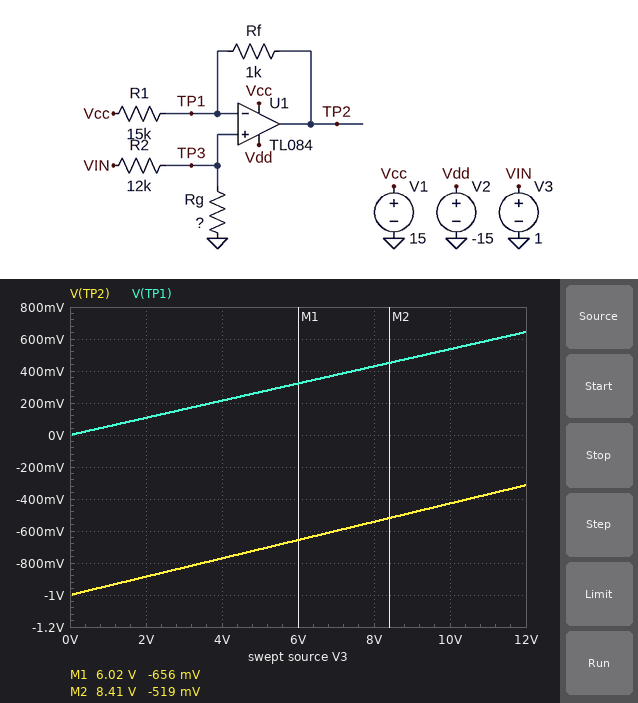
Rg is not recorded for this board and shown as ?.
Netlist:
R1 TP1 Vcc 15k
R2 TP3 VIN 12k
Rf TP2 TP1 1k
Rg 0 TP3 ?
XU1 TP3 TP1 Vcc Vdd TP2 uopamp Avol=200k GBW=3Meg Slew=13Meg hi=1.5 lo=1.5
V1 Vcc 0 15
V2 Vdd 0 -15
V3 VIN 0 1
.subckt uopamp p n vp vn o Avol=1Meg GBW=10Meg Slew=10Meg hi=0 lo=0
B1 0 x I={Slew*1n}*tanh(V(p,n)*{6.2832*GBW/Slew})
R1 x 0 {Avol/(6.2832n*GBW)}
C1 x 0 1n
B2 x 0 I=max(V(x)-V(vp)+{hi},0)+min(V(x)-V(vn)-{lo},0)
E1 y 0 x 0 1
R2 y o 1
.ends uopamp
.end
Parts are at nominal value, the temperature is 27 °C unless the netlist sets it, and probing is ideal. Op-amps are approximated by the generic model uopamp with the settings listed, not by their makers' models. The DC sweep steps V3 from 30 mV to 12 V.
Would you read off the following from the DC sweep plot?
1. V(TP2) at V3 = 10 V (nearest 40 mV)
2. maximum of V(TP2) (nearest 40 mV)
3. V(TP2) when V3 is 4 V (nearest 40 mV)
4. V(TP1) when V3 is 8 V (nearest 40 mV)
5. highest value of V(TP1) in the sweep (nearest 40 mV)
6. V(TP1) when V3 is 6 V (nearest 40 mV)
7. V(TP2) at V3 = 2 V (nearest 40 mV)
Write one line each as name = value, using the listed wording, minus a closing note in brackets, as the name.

V(TP2) at V3 = 10 V = -440 mV
maximum of V(TP2) = -320 mV
V(TP2) when V3 is 4 V = -760 mV
V(TP1) when V3 is 8 V = 440 mV
highest value of V(TP1) in the sweep = 640 mV
V(TP1) when V3 is 6 V = 320 mV
V(TP2) at V3 = 2 V = -880 mV
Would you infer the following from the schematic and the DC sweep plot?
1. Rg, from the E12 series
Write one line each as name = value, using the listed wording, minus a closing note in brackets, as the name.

Rg, from the E12 series = 680 Ω
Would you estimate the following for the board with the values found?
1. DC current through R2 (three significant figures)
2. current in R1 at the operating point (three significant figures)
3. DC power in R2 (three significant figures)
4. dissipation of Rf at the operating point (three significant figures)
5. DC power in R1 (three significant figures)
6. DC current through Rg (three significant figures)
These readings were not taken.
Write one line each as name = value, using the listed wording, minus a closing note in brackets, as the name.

DC current through R2 = 78.9 µA
current in R1 at the operating point = 996 µA
DC power in R2 = 74.6 µW
dissipation of Rf at the operating point = 993 µW
DC power in R1 = 14.9 mW
DC current through Rg = 78.9 µA
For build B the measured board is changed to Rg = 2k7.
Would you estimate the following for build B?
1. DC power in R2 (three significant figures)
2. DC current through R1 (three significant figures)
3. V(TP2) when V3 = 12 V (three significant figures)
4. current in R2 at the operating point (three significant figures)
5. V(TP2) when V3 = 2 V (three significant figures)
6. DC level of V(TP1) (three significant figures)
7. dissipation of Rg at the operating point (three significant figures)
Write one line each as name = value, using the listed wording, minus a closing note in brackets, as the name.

DC power in R2 = 55.5 µW
DC current through R1 = 988 µA
V(TP2) when V3 = 12 V = 1.35 V
current in R2 at the operating point = 68.0 µA
V(TP2) when V3 = 2 V = -608 mV
DC level of V(TP1) = 184 mV
dissipation of Rg at the operating point = 12.5 µW
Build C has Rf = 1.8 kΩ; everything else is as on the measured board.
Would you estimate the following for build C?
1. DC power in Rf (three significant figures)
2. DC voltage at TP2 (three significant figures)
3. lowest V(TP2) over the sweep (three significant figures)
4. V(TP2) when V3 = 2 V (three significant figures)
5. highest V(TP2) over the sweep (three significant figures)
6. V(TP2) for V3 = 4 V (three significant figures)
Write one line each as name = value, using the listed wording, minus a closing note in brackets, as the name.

DC power in Rf = 1.79 mW
DC voltage at TP2 = -1.74 V
lowest V(TP2) over the sweep = -1.80 V
V(TP2) when V3 = 2 V = -1.68 V
highest V(TP2) over the sweep = -1.08 V
V(TP2) for V3 = 4 V = -1.56 V
